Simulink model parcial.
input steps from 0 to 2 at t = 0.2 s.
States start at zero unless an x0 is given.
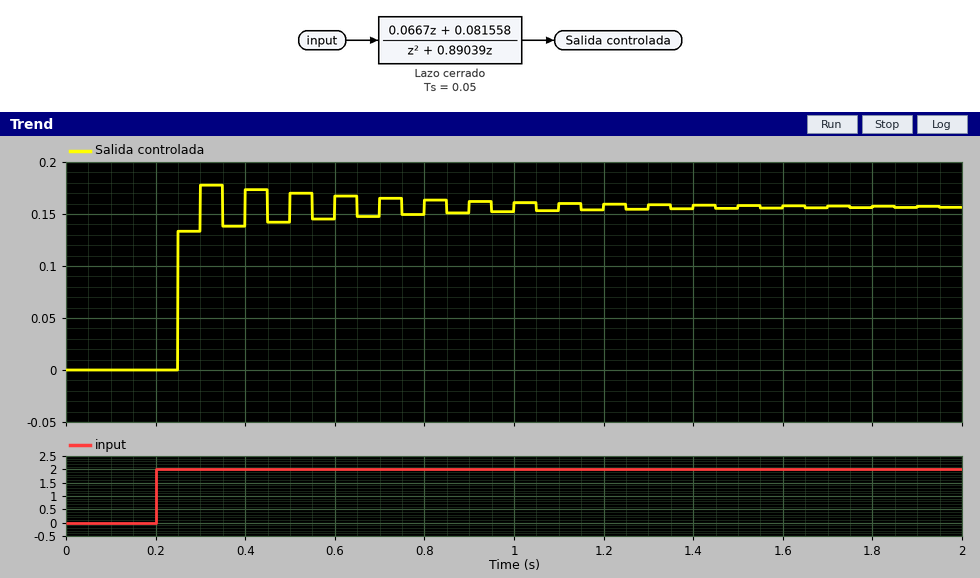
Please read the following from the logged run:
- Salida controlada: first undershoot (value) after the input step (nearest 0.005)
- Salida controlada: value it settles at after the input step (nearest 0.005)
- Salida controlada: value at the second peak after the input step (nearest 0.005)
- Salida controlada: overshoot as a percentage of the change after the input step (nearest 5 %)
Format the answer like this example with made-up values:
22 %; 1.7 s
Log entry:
0.140; 0.155; 0.175; 15 %
